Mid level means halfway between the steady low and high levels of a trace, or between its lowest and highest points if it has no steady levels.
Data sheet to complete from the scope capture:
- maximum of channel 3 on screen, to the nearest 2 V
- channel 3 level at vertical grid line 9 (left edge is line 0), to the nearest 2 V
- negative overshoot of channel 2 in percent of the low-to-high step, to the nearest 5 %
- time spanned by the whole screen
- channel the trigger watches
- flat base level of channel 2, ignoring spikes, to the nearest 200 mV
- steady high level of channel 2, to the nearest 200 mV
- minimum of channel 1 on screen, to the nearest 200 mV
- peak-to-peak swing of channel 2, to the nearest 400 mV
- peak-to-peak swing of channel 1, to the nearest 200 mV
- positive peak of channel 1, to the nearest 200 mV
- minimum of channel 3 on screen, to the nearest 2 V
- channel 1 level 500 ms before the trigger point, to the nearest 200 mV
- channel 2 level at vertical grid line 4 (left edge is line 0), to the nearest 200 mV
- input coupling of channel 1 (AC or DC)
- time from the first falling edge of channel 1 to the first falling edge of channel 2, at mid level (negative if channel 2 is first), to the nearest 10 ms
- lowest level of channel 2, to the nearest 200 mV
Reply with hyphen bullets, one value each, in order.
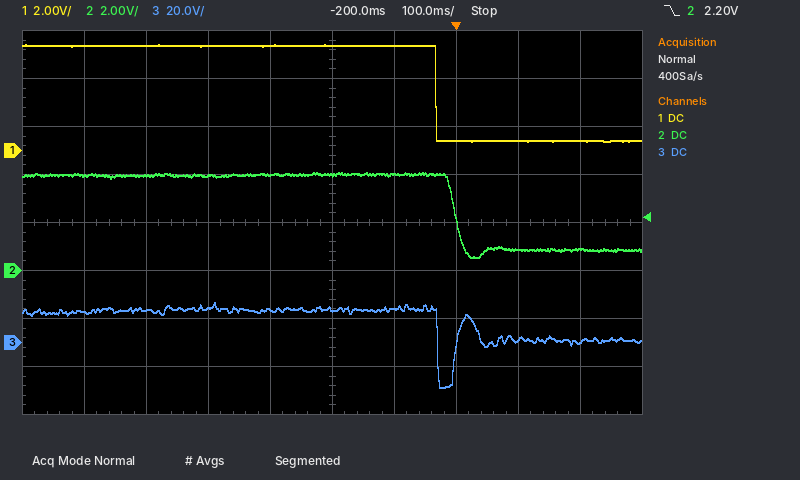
- 16 V
- 0 V
- 10 %
- 1 s
- channel 2
- 800 mV
- 4.0 V
- 400 mV
- 3.6 V
- 4.0 V
- 4.4 V
- -18 V
- 4.4 V
- 4.0 V
- DC
- +30 ms
- 600 mV
